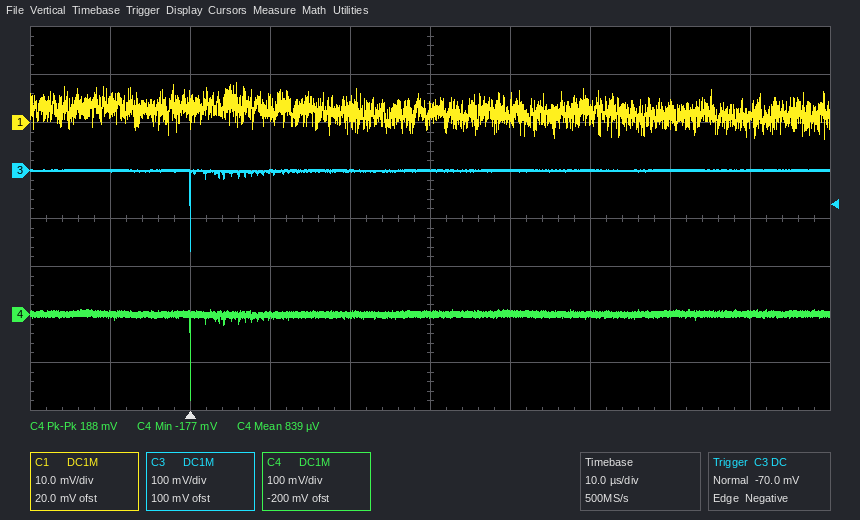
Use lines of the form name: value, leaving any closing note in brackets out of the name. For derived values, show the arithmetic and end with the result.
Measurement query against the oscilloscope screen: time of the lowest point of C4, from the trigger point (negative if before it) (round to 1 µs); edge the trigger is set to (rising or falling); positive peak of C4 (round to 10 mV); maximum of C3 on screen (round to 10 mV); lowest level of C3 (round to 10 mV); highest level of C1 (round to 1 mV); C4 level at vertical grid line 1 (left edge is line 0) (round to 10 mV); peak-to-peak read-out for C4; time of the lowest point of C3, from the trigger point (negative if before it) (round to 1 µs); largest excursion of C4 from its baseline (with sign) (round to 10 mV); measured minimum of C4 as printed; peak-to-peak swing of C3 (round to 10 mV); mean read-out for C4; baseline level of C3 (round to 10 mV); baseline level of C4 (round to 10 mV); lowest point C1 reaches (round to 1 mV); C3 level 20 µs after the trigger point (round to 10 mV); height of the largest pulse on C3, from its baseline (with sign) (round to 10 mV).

time of the lowest point of C4, from the trigger point (negative if before it): 0 µs
edge the trigger is set to: falling
positive peak of C4: 10 mV
maximum of C3 on screen: 0 mV
lowest level of C3: -170 mV
highest level of C1: 8 mV
C4 level at vertical grid line 1 (left edge is line 0): 0 mV
peak-to-peak read-out for C4: 188 mV
time of the lowest point of C3, from the trigger point (negative if before it): 0 µs
largest excursion of C4 from its baseline (with sign): -180 mV
measured minimum of C4 as printed: -177 mV
peak-to-peak swing of C3: 0 mV − (-170 mV) = 170 mV
mean read-out for C4: 839 µV
baseline level of C3: 0 mV
baseline level of C4: 0 mV
lowest point C1 reaches: -3 mV
C3 level 20 µs after the trigger point: 0 mV
height of the largest pulse on C3, from its baseline (with sign): -170 mV − (0 mV) = -170 mV
